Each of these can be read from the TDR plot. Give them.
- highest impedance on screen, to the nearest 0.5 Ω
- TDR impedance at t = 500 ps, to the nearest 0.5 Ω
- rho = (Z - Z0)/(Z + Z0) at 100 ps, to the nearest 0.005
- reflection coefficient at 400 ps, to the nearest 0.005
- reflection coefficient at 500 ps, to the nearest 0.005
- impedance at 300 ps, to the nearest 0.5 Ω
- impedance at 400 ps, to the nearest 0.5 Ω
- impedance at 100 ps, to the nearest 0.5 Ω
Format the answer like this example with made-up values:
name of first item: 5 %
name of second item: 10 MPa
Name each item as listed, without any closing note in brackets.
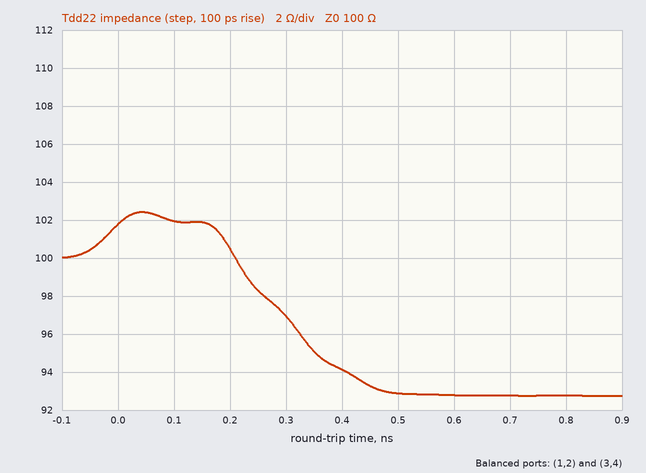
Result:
highest impedance on screen, to the nearest 0.5 Ω: 102.5 Ω
TDR impedance at t = 500 ps, to the nearest 0.5 Ω: 93.0 Ω
rho = (Z - Z0)/(Z + Z0) at 100 ps, to the nearest 0.005: +0.010
reflection coefficient at 400 ps, to the nearest 0.005: -0.030
reflection coefficient at 500 ps, to the nearest 0.005: -0.035
impedance at 300 ps, to the nearest 0.5 Ω: 97.0 Ω
impedance at 400 ps, to the nearest 0.5 Ω: 94.0 Ω
impedance at 100 ps, to the nearest 0.5 Ω: 102.0 Ω
